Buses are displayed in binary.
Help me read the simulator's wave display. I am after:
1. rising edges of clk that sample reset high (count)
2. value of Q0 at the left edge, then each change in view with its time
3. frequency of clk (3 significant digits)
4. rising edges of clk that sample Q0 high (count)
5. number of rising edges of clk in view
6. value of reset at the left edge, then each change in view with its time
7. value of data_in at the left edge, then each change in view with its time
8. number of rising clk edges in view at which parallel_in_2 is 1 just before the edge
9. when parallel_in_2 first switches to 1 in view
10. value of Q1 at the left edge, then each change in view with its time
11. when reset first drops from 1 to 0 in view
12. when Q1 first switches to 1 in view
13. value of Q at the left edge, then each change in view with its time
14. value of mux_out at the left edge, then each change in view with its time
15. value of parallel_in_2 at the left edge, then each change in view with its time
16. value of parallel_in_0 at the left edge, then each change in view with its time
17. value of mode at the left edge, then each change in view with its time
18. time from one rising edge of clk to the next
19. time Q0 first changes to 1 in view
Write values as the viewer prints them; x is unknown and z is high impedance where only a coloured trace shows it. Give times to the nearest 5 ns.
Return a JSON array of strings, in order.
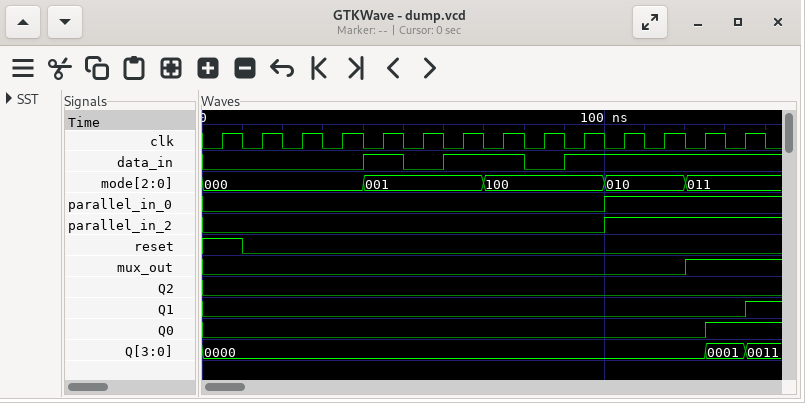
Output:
["1", "0, 1 at 125 ns", "100 MHz", "1", "14", "1, 0 at 10 ns", "0, 1 at 40 ns, 0 at 50 ns, 1 at 60 ns, 0 at 80 ns, 1 at 90 ns", "4", "100 ns", "0, 1 at 135 ns", "10 ns", "135 ns", "0000, 0001 at 125 ns, 0011 at 135 ns", "0, 1 at 120 ns", "0, 1 at 100 ns", "0, 1 at 100 ns", "000, 001 at 40 ns, 100 at 70 ns, 010 at 100 ns, 011 at 120 ns", "10 ns", "125 ns"]
